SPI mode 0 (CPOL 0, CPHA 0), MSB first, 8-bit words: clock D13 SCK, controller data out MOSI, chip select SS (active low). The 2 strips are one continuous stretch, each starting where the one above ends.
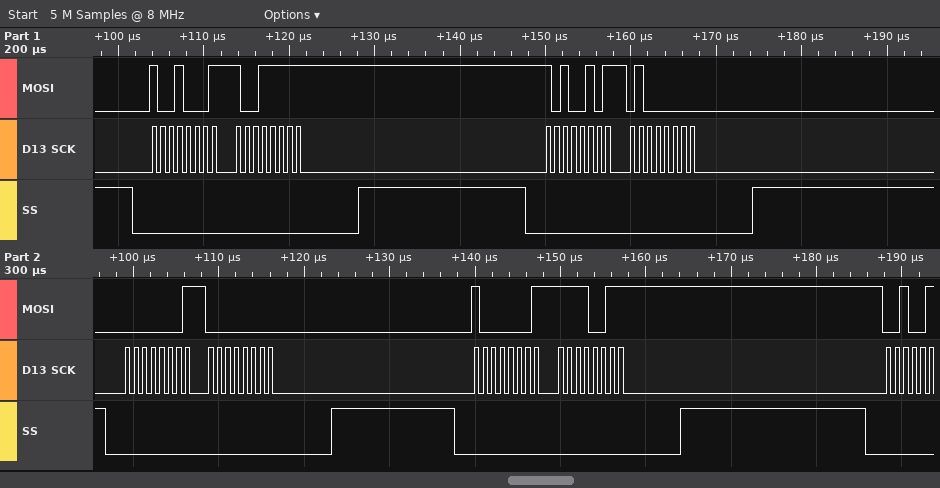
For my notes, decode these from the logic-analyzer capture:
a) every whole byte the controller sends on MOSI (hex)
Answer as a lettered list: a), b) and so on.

a) 0x91 0x9F 0xA5 0x40 0x01 0x00 0x81 0xF3
